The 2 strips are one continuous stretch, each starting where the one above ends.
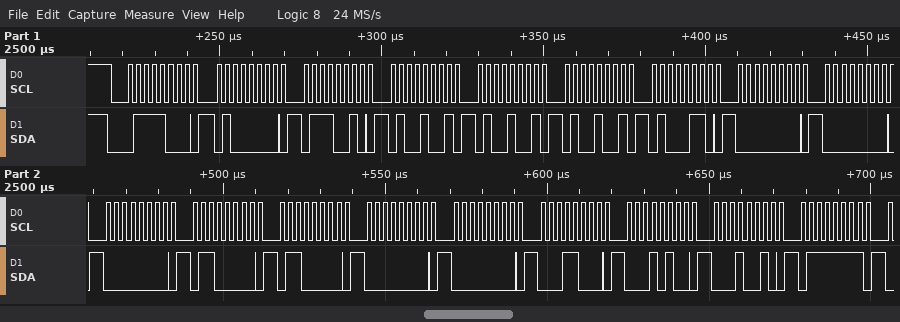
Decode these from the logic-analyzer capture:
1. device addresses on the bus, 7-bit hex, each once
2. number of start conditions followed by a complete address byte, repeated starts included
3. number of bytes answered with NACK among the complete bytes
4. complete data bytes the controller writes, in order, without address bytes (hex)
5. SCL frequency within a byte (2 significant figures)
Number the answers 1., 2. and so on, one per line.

1. 0x3C
2. 1
3. 0
4. 40 72 49 49 49 46 00 00 00 60 60 00 00 18 14 12 7F
5. 400 kHz
